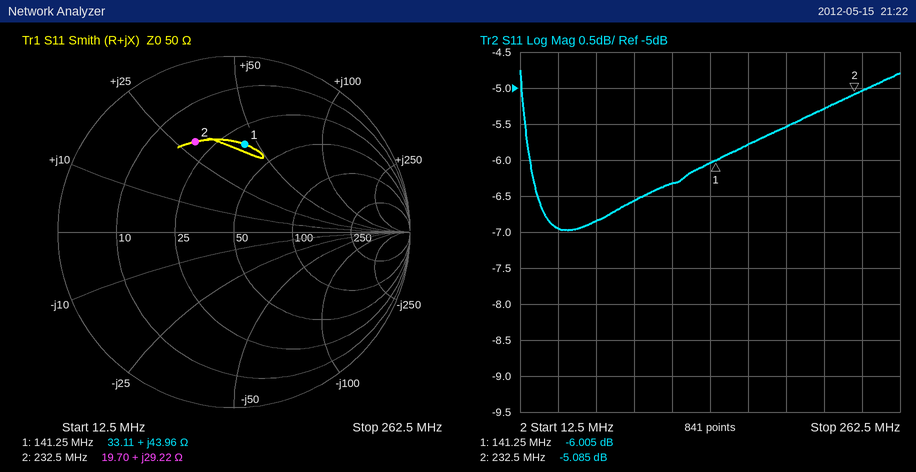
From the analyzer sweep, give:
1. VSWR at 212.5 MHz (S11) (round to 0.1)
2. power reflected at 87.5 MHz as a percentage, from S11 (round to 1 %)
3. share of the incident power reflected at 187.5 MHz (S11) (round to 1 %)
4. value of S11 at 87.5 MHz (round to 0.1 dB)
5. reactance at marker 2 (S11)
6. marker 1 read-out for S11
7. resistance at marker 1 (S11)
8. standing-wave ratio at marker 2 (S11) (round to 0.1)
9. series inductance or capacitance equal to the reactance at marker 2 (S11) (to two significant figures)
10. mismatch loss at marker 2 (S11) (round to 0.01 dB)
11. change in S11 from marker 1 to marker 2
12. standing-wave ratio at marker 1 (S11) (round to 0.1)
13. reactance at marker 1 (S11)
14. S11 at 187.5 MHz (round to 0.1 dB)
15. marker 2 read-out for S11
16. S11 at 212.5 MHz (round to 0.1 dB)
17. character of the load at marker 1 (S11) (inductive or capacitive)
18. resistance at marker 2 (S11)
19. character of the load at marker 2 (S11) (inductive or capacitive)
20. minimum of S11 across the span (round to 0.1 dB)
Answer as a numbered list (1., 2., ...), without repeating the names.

1. 3.4
2. 22 %
3. 28 %
4. -6.6 dB
5. +29.22 Ω
6. -6.005 dB
7. 33.11 Ω
8. 3.5
9. 20 nH
10. 1.61 dB
11. 0.920 dB
12. 3.0
13. +43.96 Ω
14. -5.5 dB
15. -5.085 dB
16. -5.3 dB
17. inductive
18. 19.70 Ω
19. inductive
20. -7.0 dB
